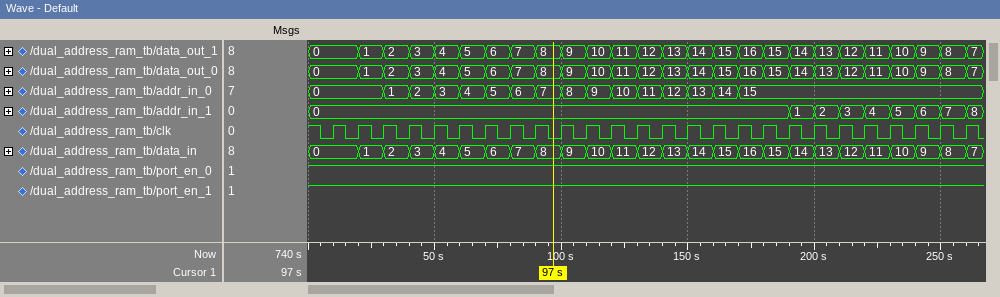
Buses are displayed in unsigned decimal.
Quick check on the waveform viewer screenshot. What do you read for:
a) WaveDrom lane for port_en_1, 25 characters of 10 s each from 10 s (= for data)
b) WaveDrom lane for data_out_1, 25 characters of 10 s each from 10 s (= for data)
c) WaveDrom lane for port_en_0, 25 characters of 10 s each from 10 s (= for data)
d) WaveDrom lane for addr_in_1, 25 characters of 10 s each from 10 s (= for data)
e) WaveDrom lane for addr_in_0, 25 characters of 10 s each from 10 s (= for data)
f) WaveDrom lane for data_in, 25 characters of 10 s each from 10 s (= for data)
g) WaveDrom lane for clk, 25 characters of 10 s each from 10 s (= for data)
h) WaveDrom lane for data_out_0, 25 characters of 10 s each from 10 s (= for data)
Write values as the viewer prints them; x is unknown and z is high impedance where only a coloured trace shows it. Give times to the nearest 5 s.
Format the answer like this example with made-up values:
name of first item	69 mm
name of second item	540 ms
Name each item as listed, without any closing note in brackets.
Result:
WaveDrom lane for port_en_1, 25 characters of 10 s each from 10 s	{name: 'port_en_1', wave: '1........................'}
WaveDrom lane for data_out_1, 25 characters of 10 s each from 10 s	{name: 'data_out_1', wave: '=========================', data: '0 1 2 3 4 5 6 7 8 9 10 11 12 13 14 15 16 15 14 13 12 11 10 9 8'}
WaveDrom lane for port_en_0, 25 characters of 10 s each from 10 s	{name: 'port_en_0', wave: '1........................'}
WaveDrom lane for addr_in_1, 25 characters of 10 s each from 10 s	{name: 'addr_in_1', wave: '=.................=======', data: '0 1 2 3 4 5 6 7'}
WaveDrom lane for addr_in_0, 25 characters of 10 s each from 10 s	{name: 'addr_in_0', wave: '=.===============........', data: '0 1 2 3 4 5 6 7 8 9 10 11 12 13 14 15'}
WaveDrom lane for data_in, 25 characters of 10 s each from 10 s	{name: 'data_in', wave: '=========================', data: '0 1 2 3 4 5 6 7 8 9 10 11 12 13 14 15 16 15 14 13 12 11 10 9 8'}
WaveDrom lane for clk, 25 characters of 10 s each from 10 s	{name: 'clk', wave: 'p........................'}
WaveDrom lane for data_out_0, 25 characters of 10 s each from 10 s	{name: 'data_out_0', wave: '=========================', data: '0 1 2 3 4 5 6 7 8 9 10 11 12 13 14 15 16 15 14 13 12 11 10 9 8'}
